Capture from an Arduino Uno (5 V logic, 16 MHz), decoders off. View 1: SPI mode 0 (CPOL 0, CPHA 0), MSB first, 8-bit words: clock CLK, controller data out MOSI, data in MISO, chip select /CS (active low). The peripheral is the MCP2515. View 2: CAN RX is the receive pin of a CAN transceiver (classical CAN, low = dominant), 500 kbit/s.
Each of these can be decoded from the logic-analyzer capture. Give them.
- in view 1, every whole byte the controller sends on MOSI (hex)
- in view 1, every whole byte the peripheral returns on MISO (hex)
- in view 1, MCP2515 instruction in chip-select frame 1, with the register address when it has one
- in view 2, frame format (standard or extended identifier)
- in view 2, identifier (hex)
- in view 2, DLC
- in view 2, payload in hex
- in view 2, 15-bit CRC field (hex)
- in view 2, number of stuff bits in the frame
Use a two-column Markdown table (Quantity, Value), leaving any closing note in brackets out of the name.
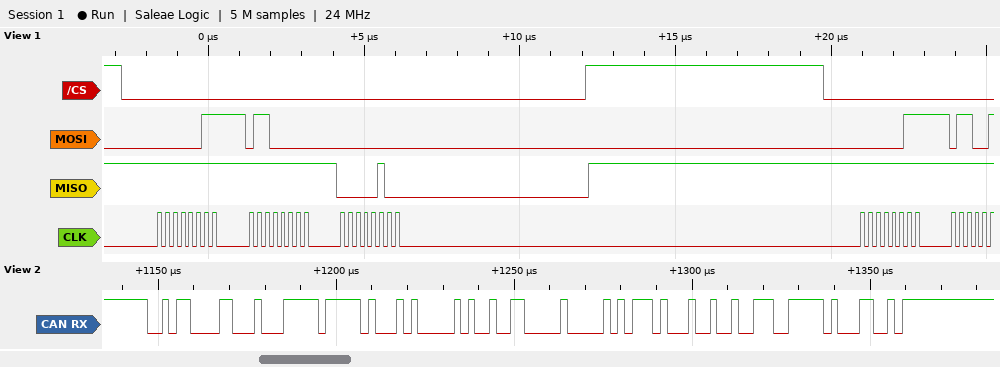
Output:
| Quantity | Value |
|---|---|
| in view 1, every whole byte the controller sends on MOSI | 03 60 00 03 |
| in view 1, every whole byte the peripheral returns on MISO | FF FF 04 FF |
| in view 1, MCP2515 instruction in chip-select frame 1, with the register address when it has one | READ 0x60 |
| in view 2, frame format | standard |
| in view 2, identifier | 0x2C3 |
| in view 2, DLC | 8 |
| in view 2, payload in hex | FF E2 81 26 00 2E 89 27 |
| in view 2, 15-bit CRC field | 0x1F8C |
| in view 2, number of stuff bits in the frame | 6 |
